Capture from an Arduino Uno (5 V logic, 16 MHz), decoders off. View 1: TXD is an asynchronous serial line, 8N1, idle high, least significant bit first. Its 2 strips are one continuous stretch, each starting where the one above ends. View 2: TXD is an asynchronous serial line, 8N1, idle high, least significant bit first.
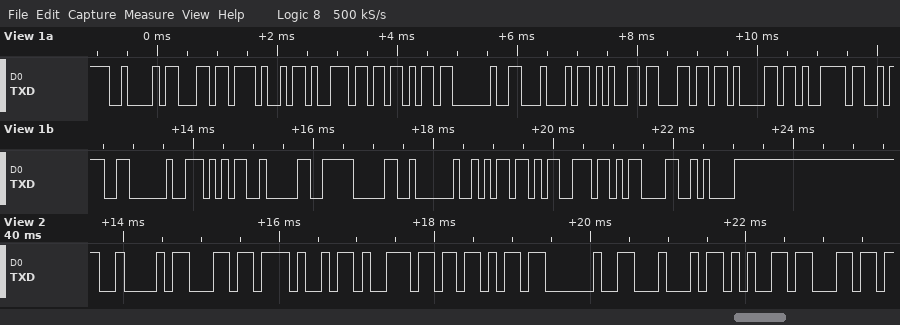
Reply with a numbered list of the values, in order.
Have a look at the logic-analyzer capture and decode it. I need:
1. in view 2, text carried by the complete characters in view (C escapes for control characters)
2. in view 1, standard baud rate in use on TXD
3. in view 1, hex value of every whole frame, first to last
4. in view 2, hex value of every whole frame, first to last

1. "Blink Del"
2. 9600 baud
3. 42 6C 69 6E 6B 20 44 65 6C 61 79 3A 20 35 30 30 20 6D 73 0D 0A
4. 42 6C 69 6E 6B 20 44 65 6C
